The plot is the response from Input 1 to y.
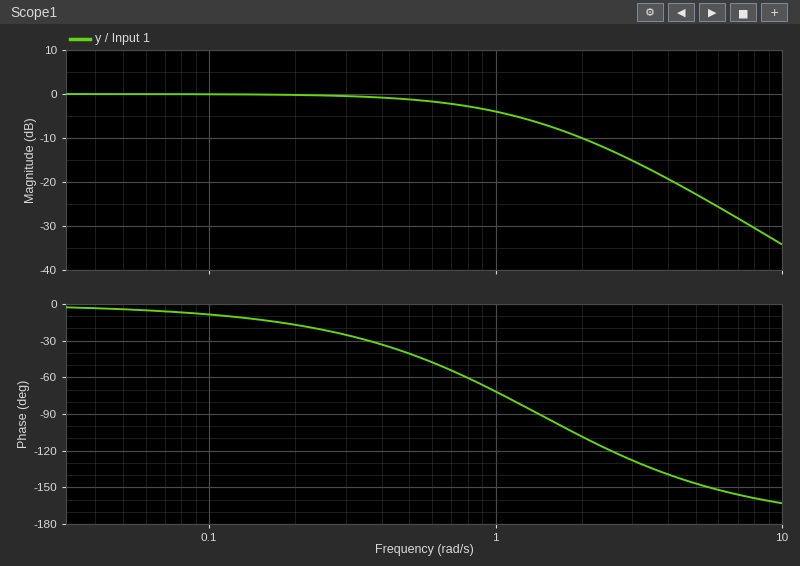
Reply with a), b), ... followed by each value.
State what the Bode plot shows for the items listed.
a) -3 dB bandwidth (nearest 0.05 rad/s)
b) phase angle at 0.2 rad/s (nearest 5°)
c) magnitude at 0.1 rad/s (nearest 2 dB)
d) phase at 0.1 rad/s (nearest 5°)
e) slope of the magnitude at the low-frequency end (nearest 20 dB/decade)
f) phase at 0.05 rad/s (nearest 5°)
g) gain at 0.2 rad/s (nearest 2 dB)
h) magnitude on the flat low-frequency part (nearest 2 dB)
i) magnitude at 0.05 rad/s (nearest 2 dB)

a) 0.85 rad/s
b) -15°
c) 0 dB
d) -10°
e) 0 dB/decade
f) -5°
g) 0 dB
h) 0 dB
i) 0 dB
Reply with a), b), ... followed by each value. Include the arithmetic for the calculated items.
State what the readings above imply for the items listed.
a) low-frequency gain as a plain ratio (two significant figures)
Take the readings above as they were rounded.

a) 10^(0 / 20) = 1.0
